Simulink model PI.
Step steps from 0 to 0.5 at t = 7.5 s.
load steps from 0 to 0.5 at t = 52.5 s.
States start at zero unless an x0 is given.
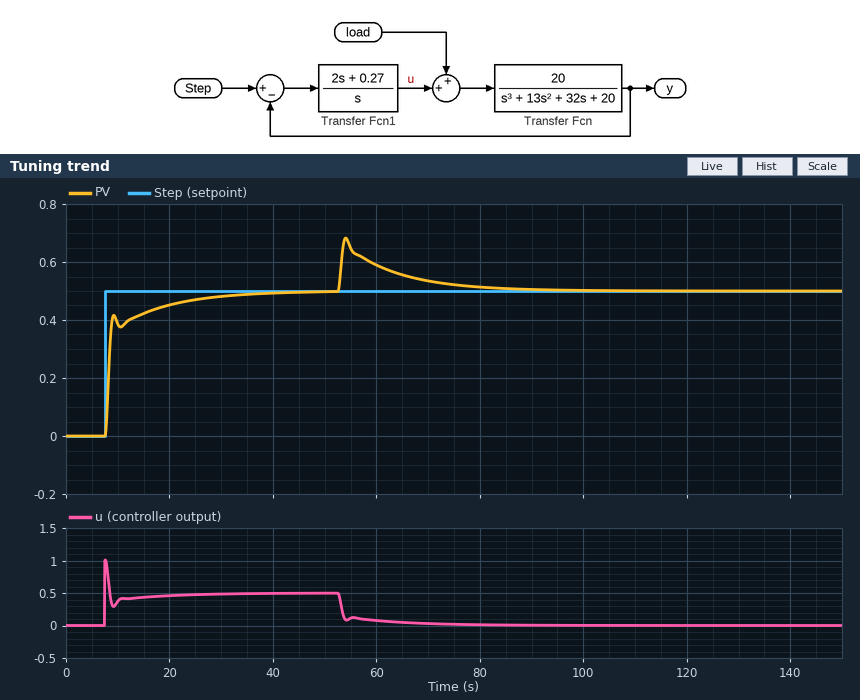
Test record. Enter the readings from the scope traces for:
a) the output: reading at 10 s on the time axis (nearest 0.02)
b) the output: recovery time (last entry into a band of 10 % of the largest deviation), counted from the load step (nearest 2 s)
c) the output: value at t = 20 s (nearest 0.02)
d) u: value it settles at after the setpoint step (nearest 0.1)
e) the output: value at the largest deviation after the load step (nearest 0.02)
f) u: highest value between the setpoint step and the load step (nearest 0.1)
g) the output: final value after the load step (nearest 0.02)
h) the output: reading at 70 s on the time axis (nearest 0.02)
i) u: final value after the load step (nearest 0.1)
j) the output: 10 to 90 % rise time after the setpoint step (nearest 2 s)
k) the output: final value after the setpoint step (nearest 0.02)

0.38
24 s
0.46
0.5
0.68
1.0
0.50
0.54
0.0
12 s
0.50
